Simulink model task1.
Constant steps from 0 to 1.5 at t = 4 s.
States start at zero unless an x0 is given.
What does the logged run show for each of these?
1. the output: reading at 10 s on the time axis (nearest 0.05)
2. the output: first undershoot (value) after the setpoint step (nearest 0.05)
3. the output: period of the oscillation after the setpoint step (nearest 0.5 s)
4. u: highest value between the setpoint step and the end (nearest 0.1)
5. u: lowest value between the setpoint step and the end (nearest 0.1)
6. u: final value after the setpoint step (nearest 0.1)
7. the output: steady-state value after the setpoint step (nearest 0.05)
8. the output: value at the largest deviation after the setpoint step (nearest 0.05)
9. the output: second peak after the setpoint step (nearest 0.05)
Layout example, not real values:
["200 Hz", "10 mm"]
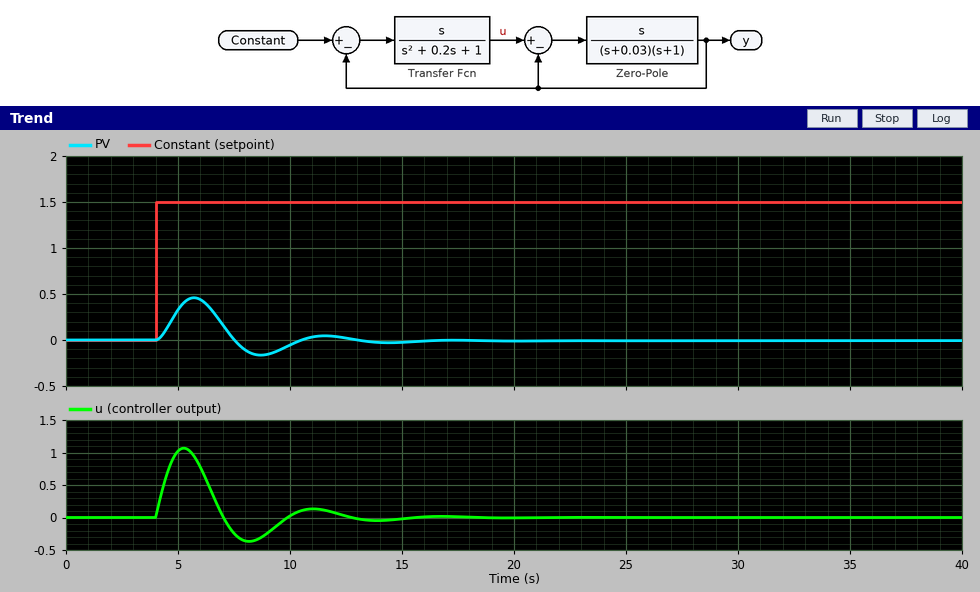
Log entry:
["-0.05", "-0.15", "6.0 s", "1.1", "-0.4", "0.0", "0.00", "0.45", "0.05"]
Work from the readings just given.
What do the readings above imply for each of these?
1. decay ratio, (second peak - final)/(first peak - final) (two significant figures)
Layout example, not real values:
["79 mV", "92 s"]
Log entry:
["0.11"]
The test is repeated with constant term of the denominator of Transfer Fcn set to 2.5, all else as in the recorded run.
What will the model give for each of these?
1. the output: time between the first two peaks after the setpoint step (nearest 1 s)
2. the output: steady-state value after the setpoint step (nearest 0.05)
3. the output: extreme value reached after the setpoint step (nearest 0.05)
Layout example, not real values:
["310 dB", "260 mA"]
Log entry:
["4 s", "0.00", "0.30"]
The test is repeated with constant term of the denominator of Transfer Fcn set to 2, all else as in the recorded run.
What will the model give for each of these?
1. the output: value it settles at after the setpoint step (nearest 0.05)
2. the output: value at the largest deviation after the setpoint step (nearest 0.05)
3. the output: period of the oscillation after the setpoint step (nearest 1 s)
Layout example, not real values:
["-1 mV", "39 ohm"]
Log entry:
["0.00", "0.35", "4 s"]
